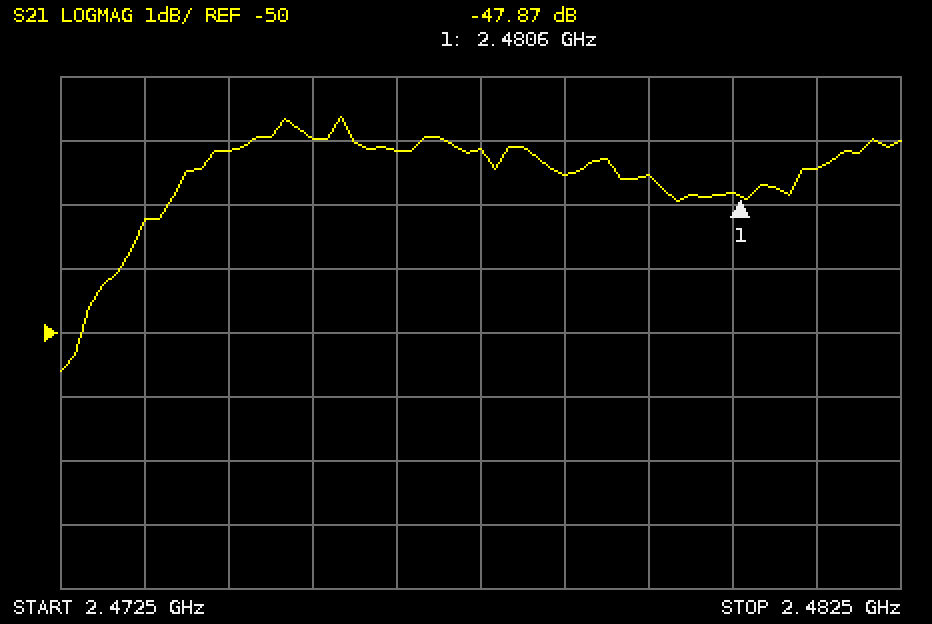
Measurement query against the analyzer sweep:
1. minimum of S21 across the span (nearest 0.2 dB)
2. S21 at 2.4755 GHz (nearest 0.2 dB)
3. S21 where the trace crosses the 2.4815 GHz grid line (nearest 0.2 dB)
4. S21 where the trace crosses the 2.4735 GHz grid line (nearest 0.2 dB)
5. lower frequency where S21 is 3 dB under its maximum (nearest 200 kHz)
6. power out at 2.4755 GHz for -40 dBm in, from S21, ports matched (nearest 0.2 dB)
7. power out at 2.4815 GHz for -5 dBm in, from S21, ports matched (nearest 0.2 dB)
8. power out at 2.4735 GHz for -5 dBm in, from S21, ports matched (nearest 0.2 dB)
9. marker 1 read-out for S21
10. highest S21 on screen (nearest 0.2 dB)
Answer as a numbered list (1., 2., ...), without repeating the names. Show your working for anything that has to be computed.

1. -50.6 dB
2. -47.0 dB
3. -47.4 dB
4. -48.2 dB
5. 2.4728 GHz
6. -40 dBm + (-47.0 dB) = -87.0 dBm
7. -5 dBm + (-47.4 dB) = -52.4 dBm
8. -5 dBm + (-48.2 dB) = -53.2 dBm
9. -47.87 dB
10. -46.6 dB
